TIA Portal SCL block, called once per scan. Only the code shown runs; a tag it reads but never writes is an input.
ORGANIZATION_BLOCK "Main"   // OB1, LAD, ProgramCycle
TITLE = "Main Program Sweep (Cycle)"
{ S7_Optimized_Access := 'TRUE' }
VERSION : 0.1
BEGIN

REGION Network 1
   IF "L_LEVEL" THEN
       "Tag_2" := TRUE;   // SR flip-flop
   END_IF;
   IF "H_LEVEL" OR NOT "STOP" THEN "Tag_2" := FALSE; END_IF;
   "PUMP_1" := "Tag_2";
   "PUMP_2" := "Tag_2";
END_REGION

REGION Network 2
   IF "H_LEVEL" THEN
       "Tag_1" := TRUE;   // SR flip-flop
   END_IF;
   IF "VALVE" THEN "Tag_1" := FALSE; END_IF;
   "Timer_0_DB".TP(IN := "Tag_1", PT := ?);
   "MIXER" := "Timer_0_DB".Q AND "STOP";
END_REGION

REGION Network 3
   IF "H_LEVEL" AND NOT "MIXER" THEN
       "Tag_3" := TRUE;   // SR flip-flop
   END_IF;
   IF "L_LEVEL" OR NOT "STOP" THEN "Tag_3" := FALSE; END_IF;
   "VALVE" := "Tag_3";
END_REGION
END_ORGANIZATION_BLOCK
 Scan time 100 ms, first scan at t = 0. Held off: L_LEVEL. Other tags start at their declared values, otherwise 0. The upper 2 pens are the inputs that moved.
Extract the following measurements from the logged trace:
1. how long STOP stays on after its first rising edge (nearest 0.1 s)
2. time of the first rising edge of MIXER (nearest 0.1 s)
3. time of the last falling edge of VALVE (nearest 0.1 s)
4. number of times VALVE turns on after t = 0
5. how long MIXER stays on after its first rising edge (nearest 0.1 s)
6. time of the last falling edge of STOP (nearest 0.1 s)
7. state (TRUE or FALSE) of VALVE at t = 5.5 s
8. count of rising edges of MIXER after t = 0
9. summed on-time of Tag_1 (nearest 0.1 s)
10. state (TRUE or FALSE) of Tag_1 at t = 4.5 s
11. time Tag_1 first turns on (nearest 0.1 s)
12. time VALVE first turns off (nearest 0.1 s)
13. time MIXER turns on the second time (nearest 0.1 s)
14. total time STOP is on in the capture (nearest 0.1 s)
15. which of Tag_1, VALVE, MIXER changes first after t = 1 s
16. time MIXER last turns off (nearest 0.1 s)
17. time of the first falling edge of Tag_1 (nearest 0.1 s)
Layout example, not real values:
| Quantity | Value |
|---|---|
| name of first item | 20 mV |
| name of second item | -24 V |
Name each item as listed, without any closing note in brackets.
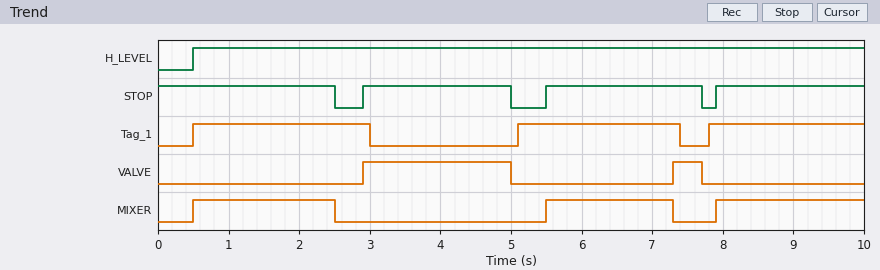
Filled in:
| Quantity | Value |
|---|---|
| how long STOP stays on after its first rising edge | 2.1 s |
| time of the first rising edge of MIXER | 0.5 s |
| time of the last falling edge of VALVE | 7.7 s |
| number of times VALVE turns on after t = 0 | 2 |
| how long MIXER stays on after its first rising edge | 2.0 s |
| time of the last falling edge of STOP | 7.7 s |
| state (TRUE or FALSE) of VALVE at t = 5.5 s | FALSE |
| count of rising edges of MIXER after t = 0 | 3 |
| summed on-time of Tag_1 | 7.0 s |
| state (TRUE or FALSE) of Tag_1 at t = 4.5 s | FALSE |
| time Tag_1 first turns on | 0.5 s |
| time VALVE first turns off | 5.0 s |
| time MIXER turns on the second time | 5.5 s |
| total time STOP is on in the capture | 8.9 s |
| which of Tag_1, VALVE, MIXER changes first after t = 1 s | MIXER |
| time MIXER last turns off | 7.3 s |
| time of the first falling edge of Tag_1 | 3.0 s |
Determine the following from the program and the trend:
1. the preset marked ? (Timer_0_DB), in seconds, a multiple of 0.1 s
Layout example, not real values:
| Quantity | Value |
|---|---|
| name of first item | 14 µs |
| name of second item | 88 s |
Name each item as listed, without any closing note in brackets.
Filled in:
| Quantity | Value |
|---|---|
| the preset marked ? (Timer_0_DB), in seconds, a multiple of 0.1 s | 2.2 s |
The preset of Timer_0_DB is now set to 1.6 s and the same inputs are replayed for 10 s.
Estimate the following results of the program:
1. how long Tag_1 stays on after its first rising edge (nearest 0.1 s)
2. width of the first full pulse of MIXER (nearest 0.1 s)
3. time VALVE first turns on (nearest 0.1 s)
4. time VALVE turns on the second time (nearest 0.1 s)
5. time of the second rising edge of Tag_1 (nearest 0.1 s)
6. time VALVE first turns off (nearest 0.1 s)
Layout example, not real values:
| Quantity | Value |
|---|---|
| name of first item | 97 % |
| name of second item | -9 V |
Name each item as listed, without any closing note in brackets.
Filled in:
| Quantity | Value |
|---|---|
| how long Tag_1 stays on after its first rising edge | 1.7 s |
| width of the first full pulse of MIXER | 1.6 s |
| time VALVE first turns on | 2.1 s |
| time VALVE turns on the second time | 4.2 s |
| time of the second rising edge of Tag_1 | 2.6 s |
| time VALVE first turns off | 2.5 s |
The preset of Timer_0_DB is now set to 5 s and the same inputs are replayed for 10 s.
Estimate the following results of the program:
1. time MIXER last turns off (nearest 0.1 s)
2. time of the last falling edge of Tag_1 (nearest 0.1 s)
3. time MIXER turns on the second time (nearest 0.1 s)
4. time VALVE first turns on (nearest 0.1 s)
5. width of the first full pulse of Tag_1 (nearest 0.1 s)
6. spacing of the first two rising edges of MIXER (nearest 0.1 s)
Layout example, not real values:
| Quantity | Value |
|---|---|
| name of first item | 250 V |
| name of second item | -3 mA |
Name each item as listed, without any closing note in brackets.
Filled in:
| Quantity | Value |
|---|---|
| time MIXER last turns off | 5.0 s |
| time of the last falling edge of Tag_1 | 5.6 s |
| time MIXER turns on the second time | 2.9 s |
| time VALVE first turns on | 5.5 s |
| width of the first full pulse of Tag_1 | 5.1 s |
| spacing of the first two rising edges of MIXER | 2.4 s |
